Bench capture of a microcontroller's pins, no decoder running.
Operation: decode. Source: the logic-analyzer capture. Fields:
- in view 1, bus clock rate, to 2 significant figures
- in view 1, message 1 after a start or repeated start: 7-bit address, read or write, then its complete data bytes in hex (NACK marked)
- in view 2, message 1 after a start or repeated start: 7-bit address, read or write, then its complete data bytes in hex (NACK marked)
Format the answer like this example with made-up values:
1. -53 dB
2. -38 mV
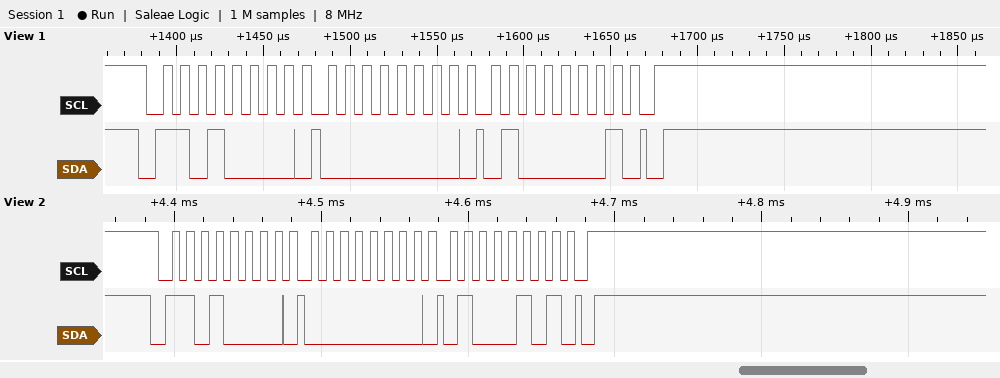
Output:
1. 100 kHz
2. 0x68 write: 00 41
3. 0x68 write: 00 45
